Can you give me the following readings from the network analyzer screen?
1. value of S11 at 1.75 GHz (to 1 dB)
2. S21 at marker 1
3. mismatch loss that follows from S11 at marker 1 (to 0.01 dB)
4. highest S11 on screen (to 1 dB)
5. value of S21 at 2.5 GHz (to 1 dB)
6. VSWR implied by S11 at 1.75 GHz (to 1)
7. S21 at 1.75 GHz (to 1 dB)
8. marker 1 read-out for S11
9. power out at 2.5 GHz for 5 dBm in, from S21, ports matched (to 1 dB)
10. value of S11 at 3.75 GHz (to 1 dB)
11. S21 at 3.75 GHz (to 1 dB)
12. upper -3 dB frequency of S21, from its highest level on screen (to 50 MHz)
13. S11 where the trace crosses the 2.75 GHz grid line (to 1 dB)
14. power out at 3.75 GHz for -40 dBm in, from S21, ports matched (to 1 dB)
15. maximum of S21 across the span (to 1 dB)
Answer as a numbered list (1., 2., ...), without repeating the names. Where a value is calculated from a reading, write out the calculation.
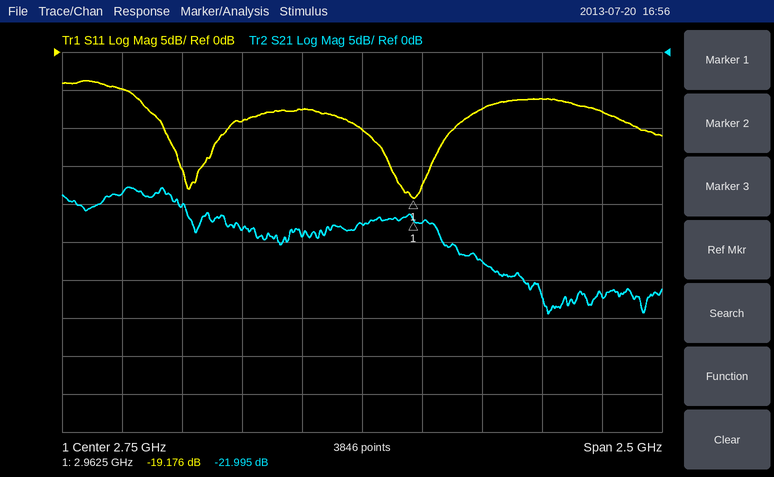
1. -5 dB
2. -21.995 dB
3. −10 log10(1 − 10^(-19.176/10)) ≈ 0.05 dB
4. -4 dB
5. -24 dB
6. |Γ| = 10^(-5/20) = 0.5623; VSWR = (1 + 0.5623)/(1 − 0.5623) ≈ 4
7. -19 dB
8. -19.176 dB
9. 5 dBm + (-24 dB) = -19 dBm
10. -8 dB
11. -32 dB
12. 2.00 GHz
13. -10 dB
14. -40 dBm + (-32 dB) = -72 dBm
15. -18 dB
